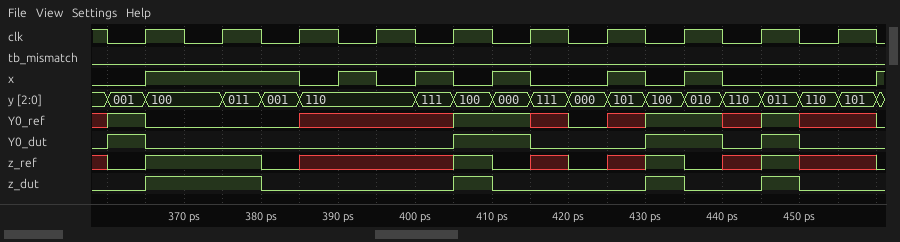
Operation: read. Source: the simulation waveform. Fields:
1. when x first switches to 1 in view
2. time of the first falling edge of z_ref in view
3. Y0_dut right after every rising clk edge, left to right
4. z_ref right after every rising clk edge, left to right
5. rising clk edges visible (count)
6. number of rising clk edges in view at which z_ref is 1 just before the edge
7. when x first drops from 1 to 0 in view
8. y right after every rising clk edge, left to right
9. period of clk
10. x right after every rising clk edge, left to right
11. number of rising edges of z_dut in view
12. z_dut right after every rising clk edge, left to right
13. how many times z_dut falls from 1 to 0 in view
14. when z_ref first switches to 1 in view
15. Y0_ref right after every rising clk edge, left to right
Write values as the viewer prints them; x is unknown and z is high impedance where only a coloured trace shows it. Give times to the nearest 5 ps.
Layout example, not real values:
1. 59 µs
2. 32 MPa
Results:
1. 365 ps
2. 380 ps
3. 0 0 0 0 1 0 0 1 1 0
4. 1 1 x x 1 x x 0 1 x
5. 10
6. 2
7. 385 ps
8. 100, 011, 110, 110, 100, 111, 101, 010, 011, 101
9. 10 ps
10. 1 1 0 0 0 0 1 1 0 0
11. 4
12. 1 1 0 0 1 0 0 0 1 0
13. 4
14. 365 ps
15. 0 0 x x 1 x x 1 1 x
